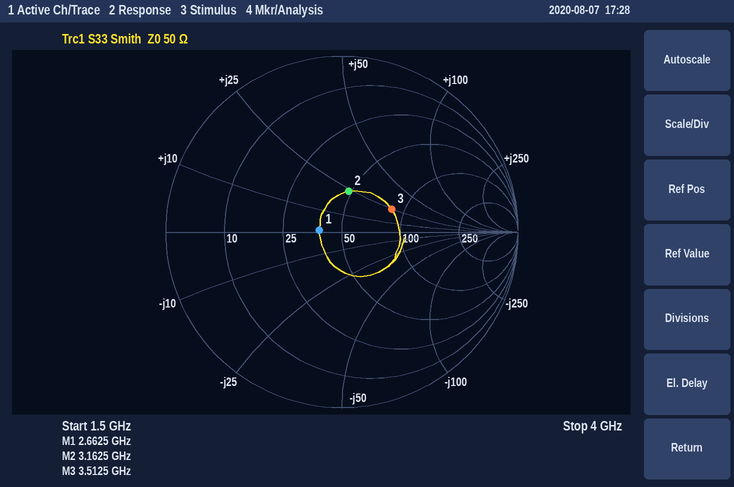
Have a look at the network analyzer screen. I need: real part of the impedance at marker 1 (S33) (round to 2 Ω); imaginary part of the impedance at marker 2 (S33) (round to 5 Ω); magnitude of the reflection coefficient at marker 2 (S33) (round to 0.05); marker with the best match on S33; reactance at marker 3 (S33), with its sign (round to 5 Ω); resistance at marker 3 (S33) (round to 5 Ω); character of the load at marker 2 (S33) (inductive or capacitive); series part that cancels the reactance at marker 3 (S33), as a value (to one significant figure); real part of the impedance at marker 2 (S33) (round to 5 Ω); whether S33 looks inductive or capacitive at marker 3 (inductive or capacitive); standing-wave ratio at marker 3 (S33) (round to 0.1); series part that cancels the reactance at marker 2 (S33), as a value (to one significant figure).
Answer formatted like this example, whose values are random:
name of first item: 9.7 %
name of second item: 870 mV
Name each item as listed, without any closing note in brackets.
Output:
real part of the impedance at marker 1 (S33): 38 Ω
imaginary part of the impedance at marker 2 (S33): +25 Ω
magnitude of the reflection coefficient at marker 2 (S33): 0.25
marker with the best match on S33: marker 1
reactance at marker 3 (S33), with its sign: +25 Ω
resistance at marker 3 (S33): 85 Ω
character of the load at marker 2 (S33): inductive
series part that cancels the reactance at marker 3 (S33), as a value: 2 pF
real part of the impedance at marker 2 (S33): 50 Ω
whether S33 looks inductive or capacitive at marker 3: inductive
standing-wave ratio at marker 3 (S33): 1.9
series part that cancels the reactance at marker 2 (S33), as a value: 2 pF
